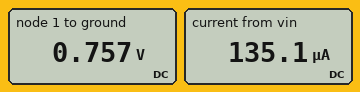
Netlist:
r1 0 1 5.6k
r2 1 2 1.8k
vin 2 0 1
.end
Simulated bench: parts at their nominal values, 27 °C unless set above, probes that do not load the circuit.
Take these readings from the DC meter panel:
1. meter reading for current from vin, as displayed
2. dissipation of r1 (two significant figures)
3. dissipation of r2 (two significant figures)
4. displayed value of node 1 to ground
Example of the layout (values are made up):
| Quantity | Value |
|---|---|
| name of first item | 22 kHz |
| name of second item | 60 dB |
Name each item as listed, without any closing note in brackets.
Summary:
| Quantity | Value |
|---|---|
| meter reading for current from vin, as displayed | 135.1 µA |
| dissipation of r1 | 100 µW |
| dissipation of r2 | 33 µW |
| displayed value of node 1 to ground | 0.757 V |
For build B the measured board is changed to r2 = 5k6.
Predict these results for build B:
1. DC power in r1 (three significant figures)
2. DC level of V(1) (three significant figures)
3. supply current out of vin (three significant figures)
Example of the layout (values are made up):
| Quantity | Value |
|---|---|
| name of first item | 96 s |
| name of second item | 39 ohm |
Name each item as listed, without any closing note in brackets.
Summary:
| Quantity | Value |
|---|---|
| DC power in r1 | 44.6 µW |
| DC level of V(1) | 500 mV |
| supply current out of vin | 89.3 µA |
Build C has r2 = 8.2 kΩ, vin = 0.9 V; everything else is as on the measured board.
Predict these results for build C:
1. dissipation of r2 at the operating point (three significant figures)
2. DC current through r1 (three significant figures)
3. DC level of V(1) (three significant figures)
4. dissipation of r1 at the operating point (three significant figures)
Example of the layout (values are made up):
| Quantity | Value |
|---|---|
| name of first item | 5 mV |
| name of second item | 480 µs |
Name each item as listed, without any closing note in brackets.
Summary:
| Quantity | Value |
|---|---|
| dissipation of r2 at the operating point | 34.9 µW |
| DC current through r1 | 65.2 µA |
| DC level of V(1) | 365 mV |
| dissipation of r1 at the operating point | 23.8 µW |
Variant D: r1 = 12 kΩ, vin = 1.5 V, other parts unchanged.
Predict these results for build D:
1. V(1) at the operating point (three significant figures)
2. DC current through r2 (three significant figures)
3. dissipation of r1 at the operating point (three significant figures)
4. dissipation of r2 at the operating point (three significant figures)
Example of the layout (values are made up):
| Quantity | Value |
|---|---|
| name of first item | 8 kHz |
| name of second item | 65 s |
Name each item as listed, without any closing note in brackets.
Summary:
| Quantity | Value |
|---|---|
| V(1) at the operating point | 1.30 V |
| DC current through r2 | 109 µA |
| dissipation of r1 at the operating point | 142 µW |
| dissipation of r2 at the operating point | 21.3 µW |
